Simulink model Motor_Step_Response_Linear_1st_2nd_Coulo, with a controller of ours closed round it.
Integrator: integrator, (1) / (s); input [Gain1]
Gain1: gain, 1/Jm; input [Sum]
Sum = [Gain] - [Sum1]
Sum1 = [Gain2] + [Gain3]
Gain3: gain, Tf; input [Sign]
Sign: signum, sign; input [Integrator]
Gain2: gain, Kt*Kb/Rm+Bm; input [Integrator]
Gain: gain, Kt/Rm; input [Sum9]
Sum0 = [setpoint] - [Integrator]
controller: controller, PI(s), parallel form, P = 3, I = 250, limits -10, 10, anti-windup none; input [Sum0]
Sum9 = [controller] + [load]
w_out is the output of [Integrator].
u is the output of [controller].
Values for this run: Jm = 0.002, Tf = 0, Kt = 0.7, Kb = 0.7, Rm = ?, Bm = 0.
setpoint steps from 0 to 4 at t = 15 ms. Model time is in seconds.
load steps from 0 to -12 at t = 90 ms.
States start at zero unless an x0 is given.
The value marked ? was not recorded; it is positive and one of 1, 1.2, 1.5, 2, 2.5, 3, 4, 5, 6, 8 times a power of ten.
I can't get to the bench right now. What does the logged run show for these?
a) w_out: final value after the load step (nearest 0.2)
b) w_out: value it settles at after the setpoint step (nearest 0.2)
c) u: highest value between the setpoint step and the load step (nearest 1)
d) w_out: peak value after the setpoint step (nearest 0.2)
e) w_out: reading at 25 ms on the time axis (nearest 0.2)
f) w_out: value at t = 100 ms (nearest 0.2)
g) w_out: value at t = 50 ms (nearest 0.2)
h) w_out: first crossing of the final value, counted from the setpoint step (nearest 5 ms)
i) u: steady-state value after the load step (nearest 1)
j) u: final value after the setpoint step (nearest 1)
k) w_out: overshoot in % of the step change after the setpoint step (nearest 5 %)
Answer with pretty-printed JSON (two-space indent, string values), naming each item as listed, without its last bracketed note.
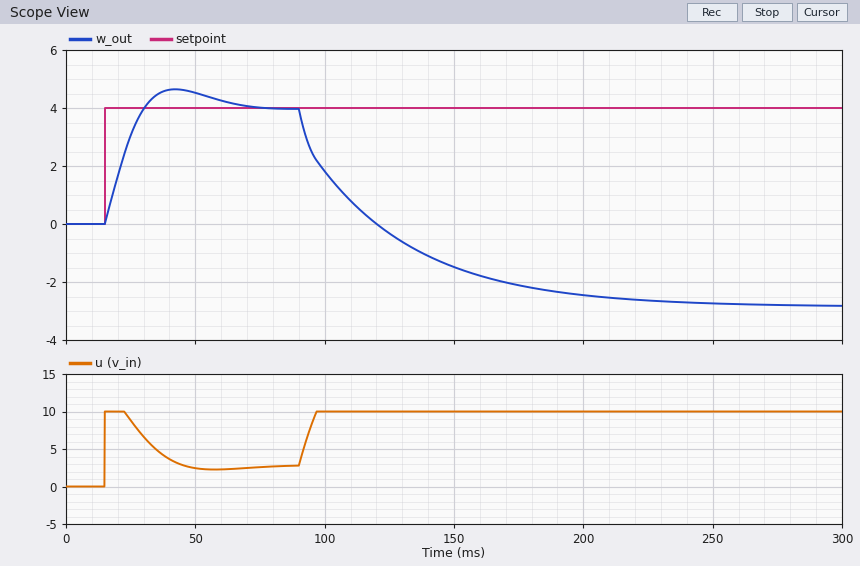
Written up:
{
  "w_out: final value after the load step": "-2.8",
  "w_out: value it settles at after the setpoint step": "4.0",
  "u: highest value between the setpoint step and the load step": "10",
  "w_out: peak value after the setpoint step": "4.6",
  "w_out: reading at 25 ms on the time axis": "3.0",
  "w_out: value at t = 100 ms": "1.8",
  "w_out: value at t = 50 ms": "4.6",
  "w_out: first crossing of the final value, counted from the setpoint step": "15 ms",
  "u: steady-state value after the load step": "10",
  "u: final value after the setpoint step": "3",
  "w_out: overshoot in % of the step change after the setpoint step": "15 %"
}
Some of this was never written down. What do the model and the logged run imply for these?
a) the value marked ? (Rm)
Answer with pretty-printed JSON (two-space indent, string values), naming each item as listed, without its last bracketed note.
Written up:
{
  "the value marked ?": "10"
}
